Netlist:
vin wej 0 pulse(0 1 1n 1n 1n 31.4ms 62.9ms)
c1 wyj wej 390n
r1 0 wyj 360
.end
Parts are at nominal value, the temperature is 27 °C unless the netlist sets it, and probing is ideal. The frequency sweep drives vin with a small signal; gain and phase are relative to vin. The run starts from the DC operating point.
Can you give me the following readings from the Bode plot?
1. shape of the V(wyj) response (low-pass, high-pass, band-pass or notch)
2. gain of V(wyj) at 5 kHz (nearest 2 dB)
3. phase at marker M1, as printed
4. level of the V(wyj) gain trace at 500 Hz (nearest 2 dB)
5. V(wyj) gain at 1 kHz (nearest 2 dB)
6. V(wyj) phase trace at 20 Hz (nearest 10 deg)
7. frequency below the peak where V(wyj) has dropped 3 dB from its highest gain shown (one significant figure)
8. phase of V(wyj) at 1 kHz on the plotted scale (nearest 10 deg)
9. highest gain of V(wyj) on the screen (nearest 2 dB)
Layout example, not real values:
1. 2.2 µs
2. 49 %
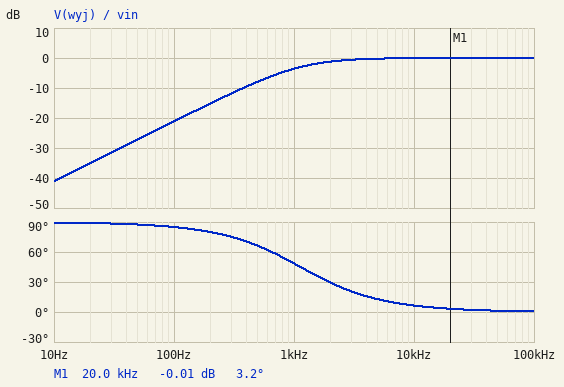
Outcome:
1. high-pass
2. 0 dB
3. 3.2 deg
4. -8 dB
5. -4 dB
6. 90 deg
7. 1 kHz
8. 50 deg
9. 0 dB
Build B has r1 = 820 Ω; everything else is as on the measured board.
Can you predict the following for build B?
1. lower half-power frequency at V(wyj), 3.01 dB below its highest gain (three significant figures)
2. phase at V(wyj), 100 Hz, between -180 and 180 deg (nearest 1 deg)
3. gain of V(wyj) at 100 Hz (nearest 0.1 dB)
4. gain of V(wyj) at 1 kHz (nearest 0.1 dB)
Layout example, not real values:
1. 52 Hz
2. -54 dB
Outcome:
1. 498 Hz
2. 79 deg
3. -14.1 dB
4. -1.0 dB
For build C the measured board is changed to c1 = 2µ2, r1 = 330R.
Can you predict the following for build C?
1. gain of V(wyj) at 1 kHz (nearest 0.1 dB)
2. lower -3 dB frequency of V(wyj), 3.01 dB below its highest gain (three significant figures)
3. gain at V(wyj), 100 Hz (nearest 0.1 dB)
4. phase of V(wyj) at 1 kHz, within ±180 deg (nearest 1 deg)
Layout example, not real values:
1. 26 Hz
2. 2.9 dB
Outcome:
1. -0.2 dB
2. 219 Hz
3. -7.6 dB
4. 12 deg
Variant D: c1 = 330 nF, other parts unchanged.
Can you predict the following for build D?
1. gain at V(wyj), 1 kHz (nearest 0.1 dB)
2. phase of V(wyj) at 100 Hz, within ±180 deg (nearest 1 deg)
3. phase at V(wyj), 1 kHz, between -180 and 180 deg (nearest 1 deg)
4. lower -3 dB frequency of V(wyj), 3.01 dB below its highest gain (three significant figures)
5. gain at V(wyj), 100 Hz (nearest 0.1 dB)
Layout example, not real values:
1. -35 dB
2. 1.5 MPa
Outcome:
1. -4.5 dB
2. 86 deg
3. 53 deg
4. 1.34 kHz
5. -22.6 dB
